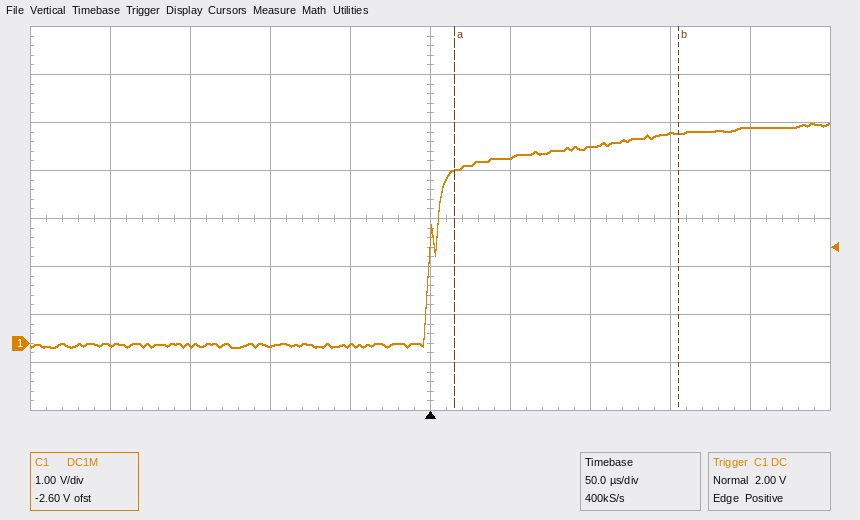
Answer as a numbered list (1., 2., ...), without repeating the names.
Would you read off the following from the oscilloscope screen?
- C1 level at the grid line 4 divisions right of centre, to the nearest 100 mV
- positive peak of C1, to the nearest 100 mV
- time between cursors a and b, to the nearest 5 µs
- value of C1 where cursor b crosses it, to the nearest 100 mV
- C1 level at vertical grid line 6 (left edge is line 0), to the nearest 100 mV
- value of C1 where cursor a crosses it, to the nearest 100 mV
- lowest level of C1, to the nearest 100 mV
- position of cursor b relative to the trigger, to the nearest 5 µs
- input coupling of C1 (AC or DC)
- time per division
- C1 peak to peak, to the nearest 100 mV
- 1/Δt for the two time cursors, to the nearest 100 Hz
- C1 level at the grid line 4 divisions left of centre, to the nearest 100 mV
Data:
1. 4.5 V
2. 4.6 V
3. 140 µs
4. 4.4 V
5. 3.9 V
6. 3.6 V
7. -100 mV
8. +155 µs
9. DC
10. 50 µs
11. 4.7 V
12. 7.1 kHz
13. 0.0 V
